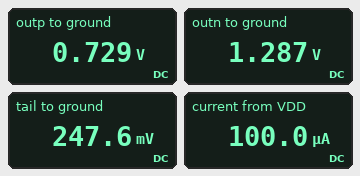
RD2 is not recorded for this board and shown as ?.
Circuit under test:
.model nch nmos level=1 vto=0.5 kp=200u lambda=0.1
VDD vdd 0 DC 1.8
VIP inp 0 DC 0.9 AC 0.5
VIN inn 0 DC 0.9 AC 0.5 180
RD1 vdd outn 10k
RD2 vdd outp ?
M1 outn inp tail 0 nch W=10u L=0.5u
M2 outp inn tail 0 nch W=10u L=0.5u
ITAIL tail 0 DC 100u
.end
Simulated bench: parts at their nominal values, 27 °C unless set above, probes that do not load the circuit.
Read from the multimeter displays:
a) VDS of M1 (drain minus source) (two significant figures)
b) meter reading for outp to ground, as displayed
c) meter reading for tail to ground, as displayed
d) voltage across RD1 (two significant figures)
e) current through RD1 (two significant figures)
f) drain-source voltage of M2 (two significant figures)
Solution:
1.0 V
0.729 V
247.6 mV
510 mV
51 µA
480 mV
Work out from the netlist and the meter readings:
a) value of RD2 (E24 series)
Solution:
22 kΩ
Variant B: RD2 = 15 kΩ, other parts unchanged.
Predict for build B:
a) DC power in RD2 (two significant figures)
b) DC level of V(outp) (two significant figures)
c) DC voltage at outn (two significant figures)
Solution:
37 µW
1.1 V
1.3 V
